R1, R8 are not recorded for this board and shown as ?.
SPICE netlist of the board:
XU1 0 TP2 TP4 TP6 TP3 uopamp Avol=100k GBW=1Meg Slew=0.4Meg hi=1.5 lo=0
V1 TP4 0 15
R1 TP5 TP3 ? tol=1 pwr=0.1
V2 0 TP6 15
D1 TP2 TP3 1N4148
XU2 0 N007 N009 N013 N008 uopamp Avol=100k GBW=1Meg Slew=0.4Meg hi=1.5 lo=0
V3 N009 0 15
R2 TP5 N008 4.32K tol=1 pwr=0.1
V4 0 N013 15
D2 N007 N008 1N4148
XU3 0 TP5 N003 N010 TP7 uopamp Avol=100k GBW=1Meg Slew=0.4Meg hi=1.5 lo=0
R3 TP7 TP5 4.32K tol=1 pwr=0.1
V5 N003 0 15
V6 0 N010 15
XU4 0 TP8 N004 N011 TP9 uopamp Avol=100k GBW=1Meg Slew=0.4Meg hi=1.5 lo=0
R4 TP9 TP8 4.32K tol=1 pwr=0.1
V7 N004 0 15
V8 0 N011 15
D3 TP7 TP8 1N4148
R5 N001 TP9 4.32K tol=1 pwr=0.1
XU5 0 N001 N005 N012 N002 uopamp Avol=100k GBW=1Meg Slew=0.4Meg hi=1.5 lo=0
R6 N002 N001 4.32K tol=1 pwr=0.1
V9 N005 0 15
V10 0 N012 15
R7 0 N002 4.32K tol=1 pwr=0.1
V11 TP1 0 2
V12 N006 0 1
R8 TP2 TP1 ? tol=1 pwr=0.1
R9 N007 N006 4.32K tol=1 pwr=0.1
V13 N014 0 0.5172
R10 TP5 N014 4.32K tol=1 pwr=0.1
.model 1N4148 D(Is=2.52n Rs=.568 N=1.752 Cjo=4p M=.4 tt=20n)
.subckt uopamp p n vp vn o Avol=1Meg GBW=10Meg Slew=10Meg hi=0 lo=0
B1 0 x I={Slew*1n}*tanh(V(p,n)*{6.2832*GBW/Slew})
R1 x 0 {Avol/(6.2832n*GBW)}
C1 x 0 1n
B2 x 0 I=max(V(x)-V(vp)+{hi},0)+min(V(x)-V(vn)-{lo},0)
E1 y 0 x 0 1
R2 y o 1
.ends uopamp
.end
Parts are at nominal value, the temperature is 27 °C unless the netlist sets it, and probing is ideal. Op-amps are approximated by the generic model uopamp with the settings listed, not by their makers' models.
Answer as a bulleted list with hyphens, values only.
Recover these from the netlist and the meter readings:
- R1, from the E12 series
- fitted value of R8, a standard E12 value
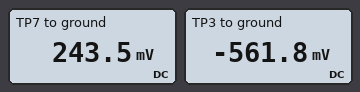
- 10 kΩ
- 3.3 kΩ
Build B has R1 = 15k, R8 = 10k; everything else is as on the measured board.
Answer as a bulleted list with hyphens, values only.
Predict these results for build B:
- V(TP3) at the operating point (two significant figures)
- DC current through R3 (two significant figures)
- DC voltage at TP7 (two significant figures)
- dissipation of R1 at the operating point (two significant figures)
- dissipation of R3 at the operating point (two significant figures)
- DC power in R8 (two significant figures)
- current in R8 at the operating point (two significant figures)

- -510 mV
- 34 µA
- 150 mV
- 17 µW
- 5.1 µW
- 400 µW
- 200 µA
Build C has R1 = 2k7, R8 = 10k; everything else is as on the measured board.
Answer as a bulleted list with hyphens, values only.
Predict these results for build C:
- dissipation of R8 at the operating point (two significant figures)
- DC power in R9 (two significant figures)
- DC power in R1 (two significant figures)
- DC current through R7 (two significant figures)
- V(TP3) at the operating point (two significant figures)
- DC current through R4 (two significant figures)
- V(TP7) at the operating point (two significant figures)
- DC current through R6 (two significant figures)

- 400 µW
- 230 µW
- 97 µW
- 3.1 mA
- -510 mV
- 3.5 mA
- 820 mV
- 3.3 mA
